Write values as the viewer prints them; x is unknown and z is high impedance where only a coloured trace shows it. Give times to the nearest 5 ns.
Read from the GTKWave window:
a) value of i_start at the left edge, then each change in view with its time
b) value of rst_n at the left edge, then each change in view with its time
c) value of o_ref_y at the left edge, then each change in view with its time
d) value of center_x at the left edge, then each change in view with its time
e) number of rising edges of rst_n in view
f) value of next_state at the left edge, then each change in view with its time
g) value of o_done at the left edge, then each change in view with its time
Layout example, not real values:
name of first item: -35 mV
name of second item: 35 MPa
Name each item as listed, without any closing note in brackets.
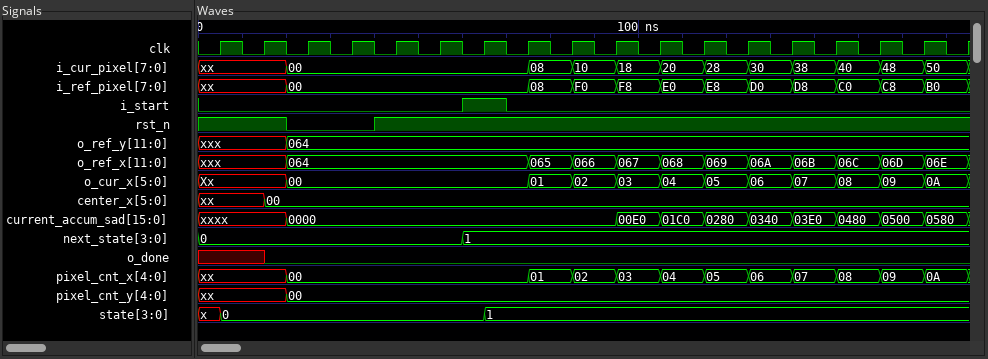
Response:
value of i_start at the left edge, then each change in view with its time: 0, 1 at 60 ns, 0 at 70 ns
value of rst_n at the left edge, then each change in view with its time: 1, 0 at 20 ns, 1 at 40 ns
value of o_ref_y at the left edge, then each change in view with its time: xxx, 064 at 20 ns
value of center_x at the left edge, then each change in view with its time: xx, 00 at 15 ns
number of rising edges of rst_n in view: 1
value of next_state at the left edge, then each change in view with its time: 0, 1 at 60 ns
value of o_done at the left edge, then each change in view with its time: x, 0 at 15 ns
